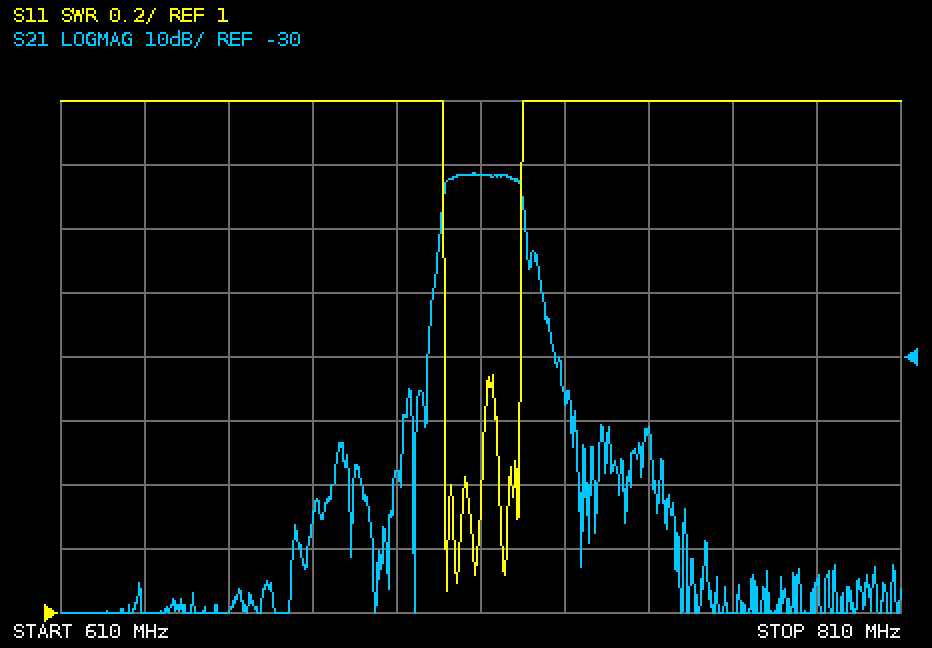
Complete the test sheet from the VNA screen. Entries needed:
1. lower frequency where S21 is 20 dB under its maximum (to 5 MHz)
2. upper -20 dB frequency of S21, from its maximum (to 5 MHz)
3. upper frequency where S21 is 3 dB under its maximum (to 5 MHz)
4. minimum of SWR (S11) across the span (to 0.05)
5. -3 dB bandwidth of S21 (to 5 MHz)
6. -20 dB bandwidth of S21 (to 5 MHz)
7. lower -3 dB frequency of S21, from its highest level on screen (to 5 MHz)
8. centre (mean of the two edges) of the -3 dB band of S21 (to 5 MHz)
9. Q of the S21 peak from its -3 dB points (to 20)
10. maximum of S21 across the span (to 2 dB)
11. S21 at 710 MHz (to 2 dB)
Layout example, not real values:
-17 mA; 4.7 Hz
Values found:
700 MHz; 725 MHz; 720 MHz; 1.05; 20 MHz; 25 MHz; 700 MHz; 710 MHz; 40; -2 dB; -2 dB
